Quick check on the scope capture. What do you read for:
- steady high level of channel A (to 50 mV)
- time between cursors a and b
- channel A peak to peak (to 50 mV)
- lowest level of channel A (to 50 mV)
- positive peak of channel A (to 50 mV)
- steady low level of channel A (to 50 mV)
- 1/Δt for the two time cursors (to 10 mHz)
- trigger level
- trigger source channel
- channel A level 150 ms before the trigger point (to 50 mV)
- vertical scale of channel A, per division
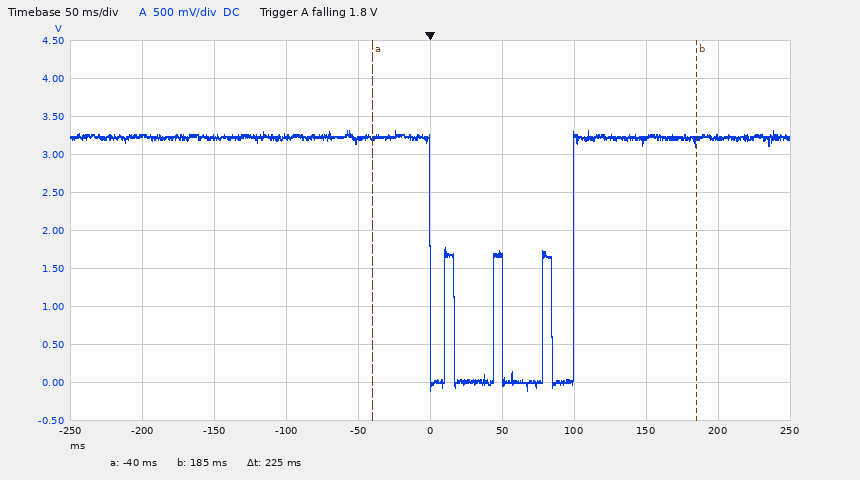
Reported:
3.25 V
225 ms
3.40 V
-100 mV
3.30 V
0 mV
4.44 Hz
1.8 V
channel A
3.25 V
500 mV
